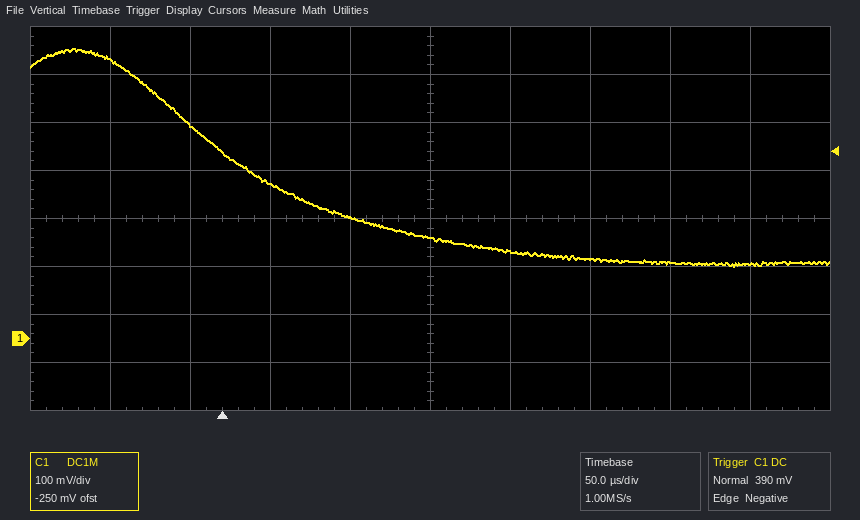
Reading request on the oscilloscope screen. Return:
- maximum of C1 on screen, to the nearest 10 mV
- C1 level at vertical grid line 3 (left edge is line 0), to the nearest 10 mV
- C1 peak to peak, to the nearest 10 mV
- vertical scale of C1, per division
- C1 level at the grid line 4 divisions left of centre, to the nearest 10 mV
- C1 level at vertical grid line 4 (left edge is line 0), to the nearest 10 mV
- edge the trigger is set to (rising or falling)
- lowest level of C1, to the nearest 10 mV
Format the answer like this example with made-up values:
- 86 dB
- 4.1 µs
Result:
- 600 mV
- 320 mV
- 450 mV
- 100 mV
- 580 mV
- 250 mV
- falling
- 150 mV
